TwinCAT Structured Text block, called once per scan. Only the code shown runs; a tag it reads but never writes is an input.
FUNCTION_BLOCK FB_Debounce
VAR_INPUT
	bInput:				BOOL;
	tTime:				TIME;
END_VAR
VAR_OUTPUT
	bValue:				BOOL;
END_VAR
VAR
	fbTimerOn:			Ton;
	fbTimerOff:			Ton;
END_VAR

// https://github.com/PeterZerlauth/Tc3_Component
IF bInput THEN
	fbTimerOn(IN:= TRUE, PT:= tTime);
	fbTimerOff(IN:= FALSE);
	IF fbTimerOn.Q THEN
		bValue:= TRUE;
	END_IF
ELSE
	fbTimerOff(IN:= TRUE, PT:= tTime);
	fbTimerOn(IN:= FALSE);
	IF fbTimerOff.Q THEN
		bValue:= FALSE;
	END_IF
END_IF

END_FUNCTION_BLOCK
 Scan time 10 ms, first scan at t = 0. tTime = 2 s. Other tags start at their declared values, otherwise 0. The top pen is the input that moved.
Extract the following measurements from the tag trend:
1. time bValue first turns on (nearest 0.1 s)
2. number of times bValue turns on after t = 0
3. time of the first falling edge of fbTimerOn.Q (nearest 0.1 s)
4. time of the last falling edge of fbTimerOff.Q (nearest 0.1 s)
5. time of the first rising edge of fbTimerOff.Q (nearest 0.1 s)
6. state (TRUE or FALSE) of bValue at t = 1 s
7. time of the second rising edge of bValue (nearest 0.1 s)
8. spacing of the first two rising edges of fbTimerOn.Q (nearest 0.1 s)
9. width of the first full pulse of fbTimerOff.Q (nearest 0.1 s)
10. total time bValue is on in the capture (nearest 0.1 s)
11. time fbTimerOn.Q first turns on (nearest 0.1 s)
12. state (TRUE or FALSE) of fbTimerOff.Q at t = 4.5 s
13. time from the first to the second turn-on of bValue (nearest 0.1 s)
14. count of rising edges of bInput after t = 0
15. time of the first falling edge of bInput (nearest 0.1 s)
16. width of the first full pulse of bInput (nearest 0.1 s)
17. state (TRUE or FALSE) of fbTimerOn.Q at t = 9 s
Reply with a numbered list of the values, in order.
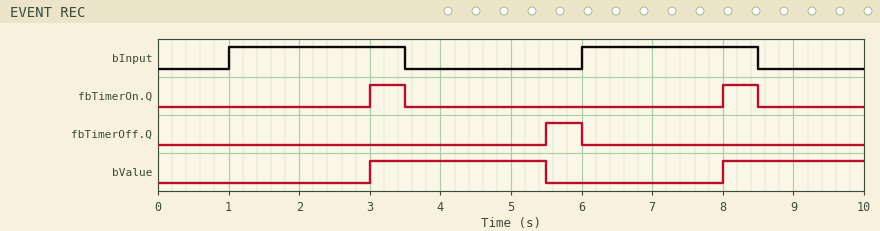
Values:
1. 3.0 s
2. 2
3. 3.5 s
4. 6.0 s
5. 5.5 s
6. FALSE
7. 8.0 s
8. 5.0 s
9. 0.5 s
10. 4.5 s
11. 3.0 s
12. FALSE
13. 5.0 s
14. 2
15. 3.5 s
16. 2.5 s
17. FALSE
